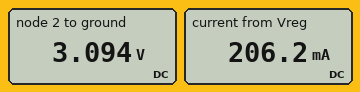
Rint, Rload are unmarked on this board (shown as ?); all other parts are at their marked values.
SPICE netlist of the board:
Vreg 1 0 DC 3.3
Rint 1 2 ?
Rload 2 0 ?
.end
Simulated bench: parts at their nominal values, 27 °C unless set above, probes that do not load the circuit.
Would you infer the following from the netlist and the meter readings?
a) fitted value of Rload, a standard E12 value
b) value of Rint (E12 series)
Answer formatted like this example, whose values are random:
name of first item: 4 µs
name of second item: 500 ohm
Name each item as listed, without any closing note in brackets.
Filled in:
fitted value of Rload, a standard E12 value: 15 Ω
value of Rint: 1 Ω
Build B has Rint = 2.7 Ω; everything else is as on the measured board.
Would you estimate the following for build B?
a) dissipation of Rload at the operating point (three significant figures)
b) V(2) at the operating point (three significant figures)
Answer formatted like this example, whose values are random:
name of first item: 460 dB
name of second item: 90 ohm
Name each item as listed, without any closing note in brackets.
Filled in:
dissipation of Rload at the operating point: 521 mW
V(2) at the operating point: 2.80 V
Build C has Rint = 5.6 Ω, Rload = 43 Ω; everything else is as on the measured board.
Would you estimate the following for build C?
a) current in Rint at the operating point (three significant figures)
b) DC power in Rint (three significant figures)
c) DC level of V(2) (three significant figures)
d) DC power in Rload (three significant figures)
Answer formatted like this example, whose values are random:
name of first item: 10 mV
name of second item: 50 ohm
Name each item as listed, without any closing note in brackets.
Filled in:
current in Rint at the operating point: 67.9 mA
DC power in Rint: 25.8 mW
DC level of V(2): 2.92 V
DC power in Rload: 198 mW
